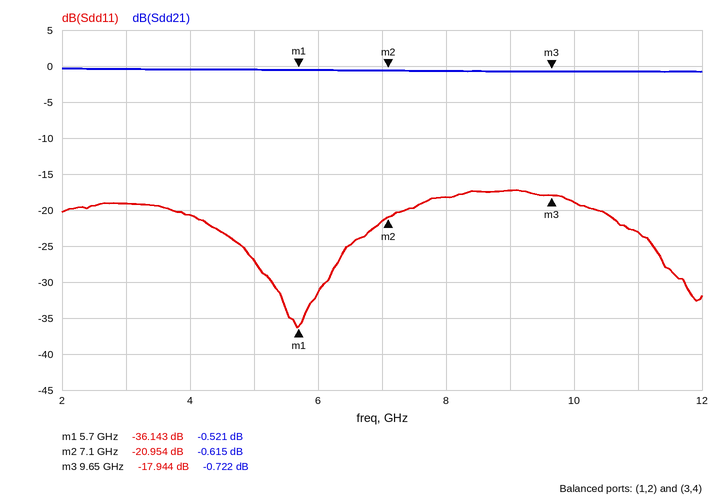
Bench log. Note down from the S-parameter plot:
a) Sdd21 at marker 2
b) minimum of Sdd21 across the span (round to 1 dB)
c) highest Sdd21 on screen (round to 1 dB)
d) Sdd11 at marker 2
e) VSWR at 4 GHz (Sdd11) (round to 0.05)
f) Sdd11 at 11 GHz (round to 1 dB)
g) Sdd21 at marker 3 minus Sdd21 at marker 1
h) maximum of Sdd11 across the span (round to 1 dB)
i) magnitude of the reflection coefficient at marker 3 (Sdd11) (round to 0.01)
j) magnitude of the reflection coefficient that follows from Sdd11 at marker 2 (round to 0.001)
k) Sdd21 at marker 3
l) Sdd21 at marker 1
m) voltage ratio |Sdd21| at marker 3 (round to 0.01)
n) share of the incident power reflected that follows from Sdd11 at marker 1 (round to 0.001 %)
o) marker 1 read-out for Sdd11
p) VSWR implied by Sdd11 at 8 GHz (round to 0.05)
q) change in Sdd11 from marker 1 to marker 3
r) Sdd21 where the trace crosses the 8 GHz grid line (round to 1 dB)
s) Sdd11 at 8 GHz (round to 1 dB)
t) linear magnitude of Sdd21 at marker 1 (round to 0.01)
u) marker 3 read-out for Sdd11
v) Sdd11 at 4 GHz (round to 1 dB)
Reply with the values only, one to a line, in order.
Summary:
-0.615 dB
-1 dB
0 dB
-20.954 dB
1.20
-23 dB
-0.201 dB
-17 dB
0.13
0.090
-0.722 dB
-0.521 dB
0.92
0.024 %
-36.143 dB
1.30
18.199 dB
-1 dB
-18 dB
0.94
-17.944 dB
-21 dB
